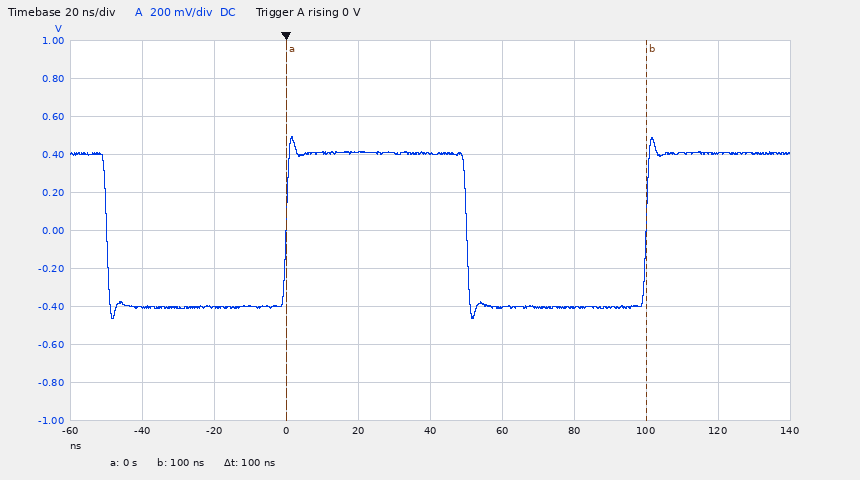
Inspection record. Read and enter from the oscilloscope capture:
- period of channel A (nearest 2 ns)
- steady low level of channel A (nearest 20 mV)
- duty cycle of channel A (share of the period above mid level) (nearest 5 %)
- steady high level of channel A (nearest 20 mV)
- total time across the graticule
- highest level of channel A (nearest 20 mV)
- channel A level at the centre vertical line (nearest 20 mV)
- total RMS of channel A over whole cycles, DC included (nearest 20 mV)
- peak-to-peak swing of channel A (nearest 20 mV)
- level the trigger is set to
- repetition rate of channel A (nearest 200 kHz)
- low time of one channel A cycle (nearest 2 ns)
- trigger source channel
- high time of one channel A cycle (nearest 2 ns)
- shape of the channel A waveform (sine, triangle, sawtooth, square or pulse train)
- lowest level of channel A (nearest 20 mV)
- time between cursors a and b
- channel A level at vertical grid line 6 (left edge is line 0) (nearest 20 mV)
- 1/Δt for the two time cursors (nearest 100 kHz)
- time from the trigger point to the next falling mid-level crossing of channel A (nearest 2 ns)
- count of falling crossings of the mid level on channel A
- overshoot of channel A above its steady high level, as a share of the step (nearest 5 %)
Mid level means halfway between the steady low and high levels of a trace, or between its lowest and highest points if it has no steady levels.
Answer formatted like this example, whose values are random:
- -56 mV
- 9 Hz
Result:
- 100 ns
- -400 mV
- 50 %
- 400 mV
- 200 ns
- 500 mV
- 400 mV
- 400 mV
- 960 mV
- 0 V
- 10.0 MHz
- 50 ns
- channel A
- 50 ns
- square
- -460 mV
- 100 ns
- -400 mV
- 10.0 MHz
- 50 ns
- 2
- 10 %
